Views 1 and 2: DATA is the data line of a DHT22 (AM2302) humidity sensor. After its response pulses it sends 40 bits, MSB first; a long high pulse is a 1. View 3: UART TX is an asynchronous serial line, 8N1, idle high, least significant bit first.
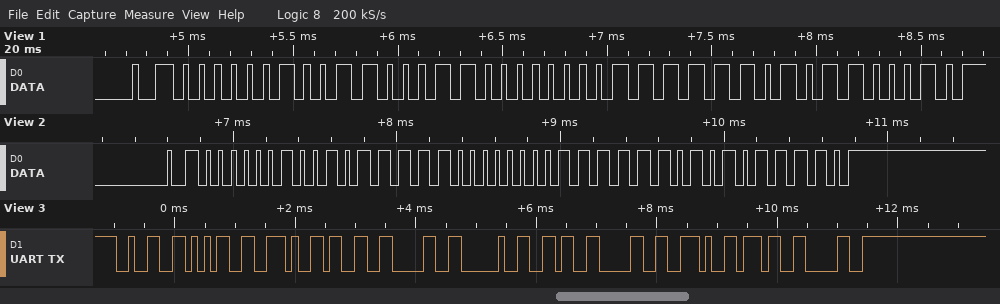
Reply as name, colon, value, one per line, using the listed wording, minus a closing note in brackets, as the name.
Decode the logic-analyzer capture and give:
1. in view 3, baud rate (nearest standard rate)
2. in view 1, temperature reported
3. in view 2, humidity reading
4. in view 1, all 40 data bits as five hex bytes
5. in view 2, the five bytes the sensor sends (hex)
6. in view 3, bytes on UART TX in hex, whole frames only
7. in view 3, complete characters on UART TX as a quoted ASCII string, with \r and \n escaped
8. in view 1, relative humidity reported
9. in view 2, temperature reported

in view 3, baud rate: 9600 baud
in view 1, temperature reported: 25.3 °C
in view 2, humidity reading: 60.7 %
in view 1, all 40 data bits as five hex bytes: 02 63 00 FD 62
in view 2, the five bytes the sensor sends: 02 5F 00 FD 5E
in view 3, bytes on UART TX in hex, whole frames only: 32 35 2E 33 30 20 36 30 2E 37 30
in view 3, complete characters on UART TX as a quoted ASCII string, with \r and \n escaped: "25.30 60.70"
in view 1, relative humidity reported: 61.1 %
in view 2, temperature reported: 25.3 °C
